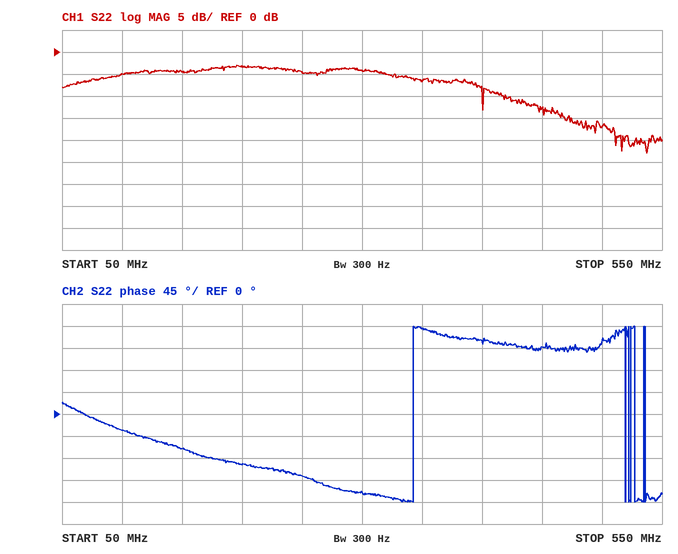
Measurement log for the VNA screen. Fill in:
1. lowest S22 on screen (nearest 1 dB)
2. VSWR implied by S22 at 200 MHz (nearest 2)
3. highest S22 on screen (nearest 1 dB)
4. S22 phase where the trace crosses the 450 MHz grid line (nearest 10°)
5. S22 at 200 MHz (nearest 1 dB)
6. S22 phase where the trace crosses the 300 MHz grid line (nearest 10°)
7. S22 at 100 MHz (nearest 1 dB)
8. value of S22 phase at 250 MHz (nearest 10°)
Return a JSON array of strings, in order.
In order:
["-23 dB", "6", "-3 dB", "140°", "-3 dB", "-160°", "-5 dB", "-130°"]
